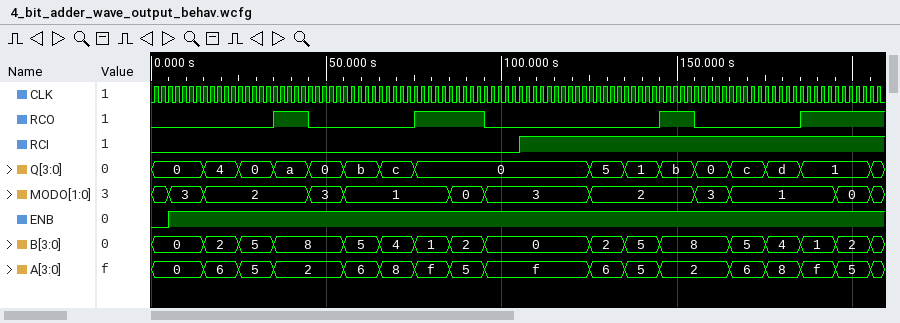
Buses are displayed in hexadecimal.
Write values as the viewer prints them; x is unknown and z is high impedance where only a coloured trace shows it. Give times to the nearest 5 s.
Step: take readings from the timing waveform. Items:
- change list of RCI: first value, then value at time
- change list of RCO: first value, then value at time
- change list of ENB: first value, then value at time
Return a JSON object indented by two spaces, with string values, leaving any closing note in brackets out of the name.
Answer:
{
  "change list of RCI: first value, then value at time": "0, 1 at 105 s",
  "change list of RCO: first value, then value at time": "0, 1 at 35 s, 0 at 45 s, 1 at 75 s, 0 at 95 s, 1 at 145 s, 0 at 155 s, 1 at 185 s",
  "change list of ENB: first value, then value at time": "0, 1 at 5 s"
}
